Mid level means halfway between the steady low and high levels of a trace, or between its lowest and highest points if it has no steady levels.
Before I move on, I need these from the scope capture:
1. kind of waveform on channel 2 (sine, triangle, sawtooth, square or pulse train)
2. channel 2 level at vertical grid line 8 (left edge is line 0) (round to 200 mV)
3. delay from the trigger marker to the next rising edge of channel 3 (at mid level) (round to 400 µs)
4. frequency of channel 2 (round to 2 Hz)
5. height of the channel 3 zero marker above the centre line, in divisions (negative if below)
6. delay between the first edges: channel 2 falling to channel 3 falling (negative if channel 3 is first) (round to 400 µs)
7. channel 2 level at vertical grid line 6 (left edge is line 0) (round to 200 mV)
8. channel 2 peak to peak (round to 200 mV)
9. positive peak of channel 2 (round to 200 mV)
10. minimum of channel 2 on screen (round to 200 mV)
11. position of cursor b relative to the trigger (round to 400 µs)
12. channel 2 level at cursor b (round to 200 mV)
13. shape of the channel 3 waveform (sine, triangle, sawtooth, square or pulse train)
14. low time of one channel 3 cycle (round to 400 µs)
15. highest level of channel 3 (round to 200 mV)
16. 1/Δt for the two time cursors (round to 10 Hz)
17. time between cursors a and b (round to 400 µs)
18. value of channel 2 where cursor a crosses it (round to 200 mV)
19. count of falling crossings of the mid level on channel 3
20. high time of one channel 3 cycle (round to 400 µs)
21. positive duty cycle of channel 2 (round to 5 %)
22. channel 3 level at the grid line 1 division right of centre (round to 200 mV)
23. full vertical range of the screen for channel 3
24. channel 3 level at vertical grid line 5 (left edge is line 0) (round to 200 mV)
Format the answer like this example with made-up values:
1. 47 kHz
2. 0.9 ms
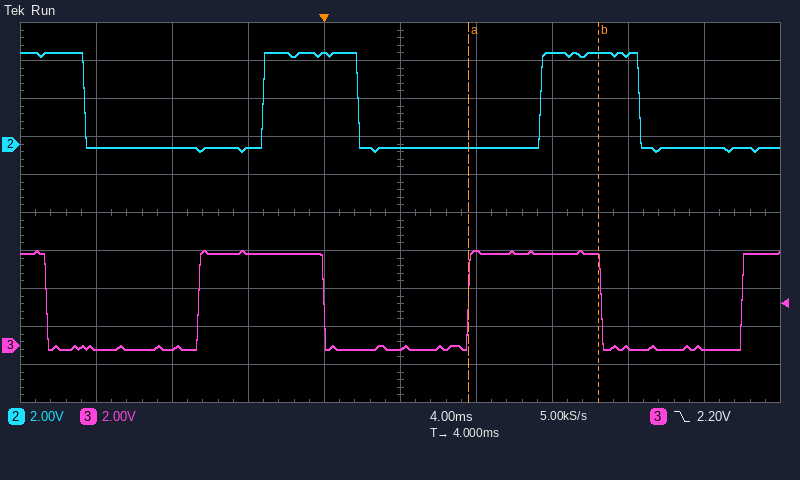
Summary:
1. pulse train
2. 4.8 V
3. 7.6 ms
4. 68 Hz
5. -3.5 div
6. -2.0 ms
7. -200 mV
8. 5.2 V
9. 4.8 V
10. -400 mV
11. +14.4 ms
12. 4.8 V
13. square
14. 7.6 ms
15. 5.0 V
16. 150 Hz
17. 6.8 ms
18. -200 mV
19. 3
20. 6.8 ms
21. 35 %
22. 5.0 V
23. 20 V
24. -200 mV
